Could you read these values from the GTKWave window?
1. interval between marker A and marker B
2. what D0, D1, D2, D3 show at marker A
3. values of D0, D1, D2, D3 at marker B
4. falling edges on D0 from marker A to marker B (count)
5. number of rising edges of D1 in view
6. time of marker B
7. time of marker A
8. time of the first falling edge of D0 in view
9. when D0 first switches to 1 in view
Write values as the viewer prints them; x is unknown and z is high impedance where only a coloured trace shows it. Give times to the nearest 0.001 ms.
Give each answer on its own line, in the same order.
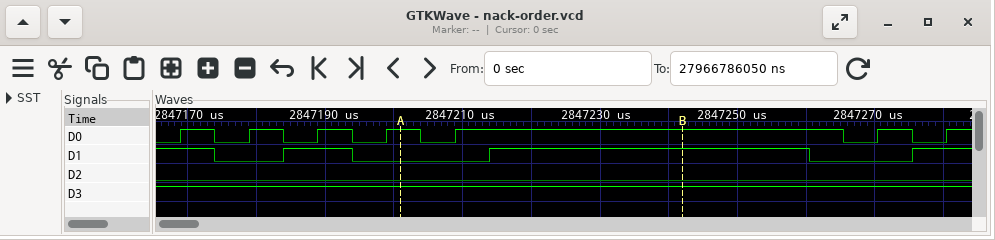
0.041 ms
D0=1, D1=0, D2=0, D3=1
D0=1, D1=1, D2=0, D3=1
1
3
2847.242 ms
2847.201 ms
2847.174 ms
2847.169 ms
